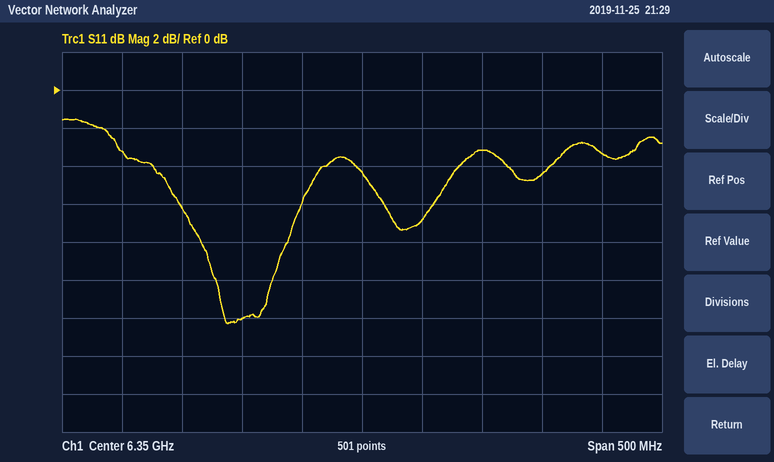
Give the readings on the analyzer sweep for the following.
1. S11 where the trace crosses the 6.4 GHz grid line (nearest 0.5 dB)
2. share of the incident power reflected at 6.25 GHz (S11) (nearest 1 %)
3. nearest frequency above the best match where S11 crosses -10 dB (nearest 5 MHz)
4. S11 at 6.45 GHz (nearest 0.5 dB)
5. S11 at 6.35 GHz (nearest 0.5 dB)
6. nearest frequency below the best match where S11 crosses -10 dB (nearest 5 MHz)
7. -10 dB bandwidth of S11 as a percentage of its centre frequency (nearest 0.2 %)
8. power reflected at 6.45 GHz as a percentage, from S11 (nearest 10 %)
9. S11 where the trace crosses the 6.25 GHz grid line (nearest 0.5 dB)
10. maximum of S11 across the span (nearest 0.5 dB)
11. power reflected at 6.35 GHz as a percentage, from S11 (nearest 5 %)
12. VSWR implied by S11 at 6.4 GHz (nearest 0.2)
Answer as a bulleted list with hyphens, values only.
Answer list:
- -7.0 dB
- 6 %
- 6.275 GHz
- -3.0 dB
- -4.5 dB
- 6.230 GHz
- 0.8 %
- 50 %
- -12.0 dB
- -1.5 dB
- 35 %
- 2.6
